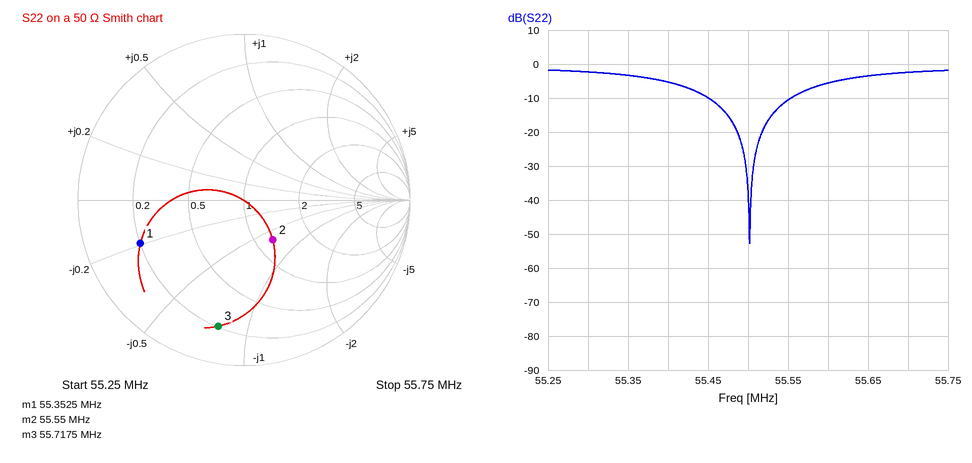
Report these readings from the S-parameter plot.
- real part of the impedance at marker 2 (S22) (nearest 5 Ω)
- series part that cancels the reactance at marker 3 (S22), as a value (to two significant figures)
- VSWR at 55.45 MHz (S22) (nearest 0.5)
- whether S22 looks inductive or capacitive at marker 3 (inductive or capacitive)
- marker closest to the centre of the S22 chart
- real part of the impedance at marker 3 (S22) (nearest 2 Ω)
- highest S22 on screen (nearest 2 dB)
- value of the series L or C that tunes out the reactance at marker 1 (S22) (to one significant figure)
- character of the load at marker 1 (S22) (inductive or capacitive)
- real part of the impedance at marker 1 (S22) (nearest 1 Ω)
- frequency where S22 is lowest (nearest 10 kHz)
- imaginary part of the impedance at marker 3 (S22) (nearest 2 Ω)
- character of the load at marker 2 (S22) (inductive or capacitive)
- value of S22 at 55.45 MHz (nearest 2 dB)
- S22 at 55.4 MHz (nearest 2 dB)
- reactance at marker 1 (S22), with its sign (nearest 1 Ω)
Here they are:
60 Ω
110 nH
2.0
capacitive
marker 2
10 Ω
-2 dB
30 nH
capacitive
10 Ω
55.50 MHz
-40 Ω
capacitive
-10 dB
-6 dB
-10 Ω
